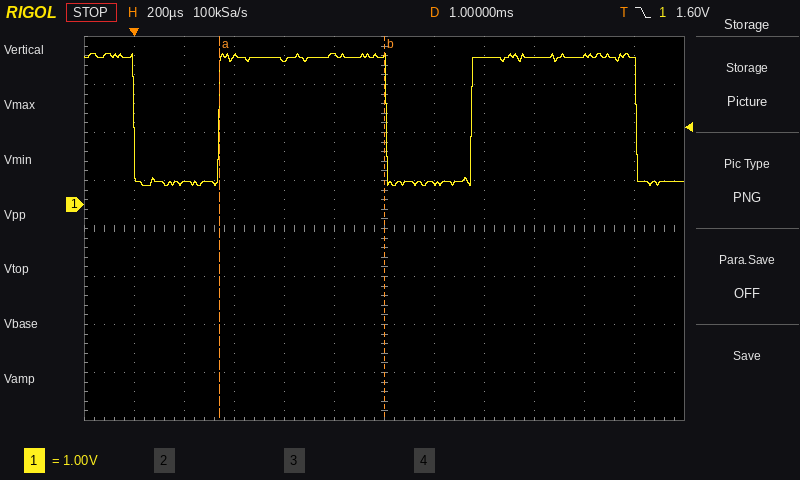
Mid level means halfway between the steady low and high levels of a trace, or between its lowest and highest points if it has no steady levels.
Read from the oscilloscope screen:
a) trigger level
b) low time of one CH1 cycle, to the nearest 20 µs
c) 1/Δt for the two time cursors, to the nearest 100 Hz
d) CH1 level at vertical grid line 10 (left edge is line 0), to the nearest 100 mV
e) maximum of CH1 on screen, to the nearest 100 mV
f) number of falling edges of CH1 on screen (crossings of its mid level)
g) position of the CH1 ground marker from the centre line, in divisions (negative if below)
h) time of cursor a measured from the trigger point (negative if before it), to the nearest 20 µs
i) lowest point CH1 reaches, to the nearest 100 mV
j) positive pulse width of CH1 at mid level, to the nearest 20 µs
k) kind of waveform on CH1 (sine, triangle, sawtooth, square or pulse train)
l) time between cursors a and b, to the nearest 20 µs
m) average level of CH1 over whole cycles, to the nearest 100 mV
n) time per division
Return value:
1.60 V
340 µs
1.5 kHz
3.1 V
3.1 V
3
+0.5 div
+340 µs
400 mV
660 µs
pulse train
660 µs
2.2 V
200 µs
